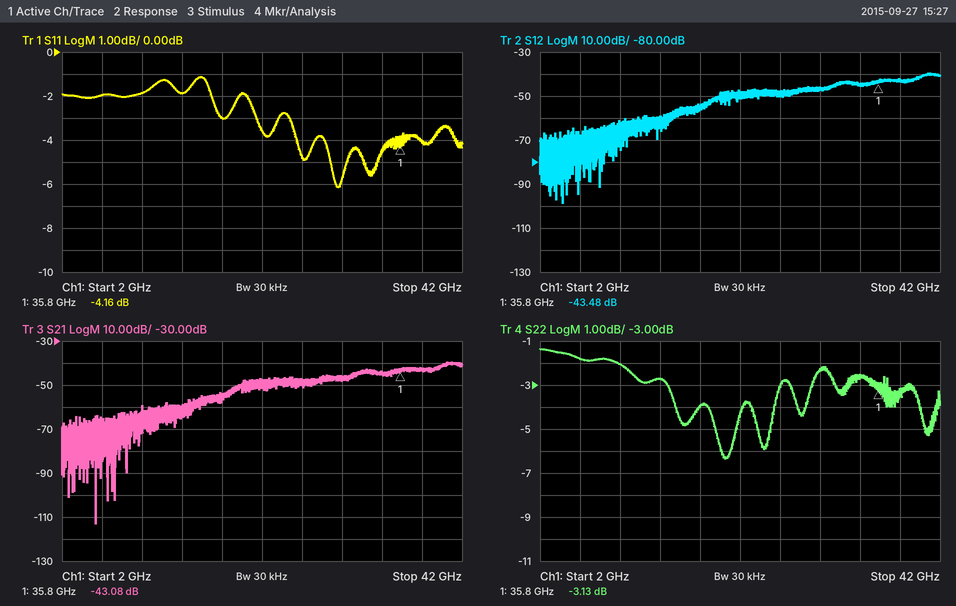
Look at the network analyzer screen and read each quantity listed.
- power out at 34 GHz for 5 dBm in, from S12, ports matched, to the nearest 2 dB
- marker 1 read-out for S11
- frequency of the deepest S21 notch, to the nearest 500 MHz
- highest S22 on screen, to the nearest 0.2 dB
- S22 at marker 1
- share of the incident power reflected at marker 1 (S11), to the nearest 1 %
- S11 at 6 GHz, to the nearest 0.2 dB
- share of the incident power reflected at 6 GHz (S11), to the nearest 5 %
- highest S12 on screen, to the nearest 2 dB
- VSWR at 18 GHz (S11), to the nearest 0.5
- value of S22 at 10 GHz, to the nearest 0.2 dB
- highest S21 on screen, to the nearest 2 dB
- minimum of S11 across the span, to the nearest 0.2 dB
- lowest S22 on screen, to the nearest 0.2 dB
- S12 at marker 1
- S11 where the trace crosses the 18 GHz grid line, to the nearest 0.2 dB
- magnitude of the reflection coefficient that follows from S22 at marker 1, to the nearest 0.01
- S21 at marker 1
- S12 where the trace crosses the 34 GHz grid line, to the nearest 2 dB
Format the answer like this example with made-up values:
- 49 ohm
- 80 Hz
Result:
- -40 dBm
- -4.16 dB
- 5.5 GHz
- -1.4 dB
- -3.13 dB
- 38 %
- -2.0 dB
- 65 %
- -40 dB
- 6.0
- -2.0 dB
- -40 dB
- -6.2 dB
- -6.4 dB
- -43.48 dB
- -3.0 dB
- 0.70
- -43.08 dB
- -44 dB
